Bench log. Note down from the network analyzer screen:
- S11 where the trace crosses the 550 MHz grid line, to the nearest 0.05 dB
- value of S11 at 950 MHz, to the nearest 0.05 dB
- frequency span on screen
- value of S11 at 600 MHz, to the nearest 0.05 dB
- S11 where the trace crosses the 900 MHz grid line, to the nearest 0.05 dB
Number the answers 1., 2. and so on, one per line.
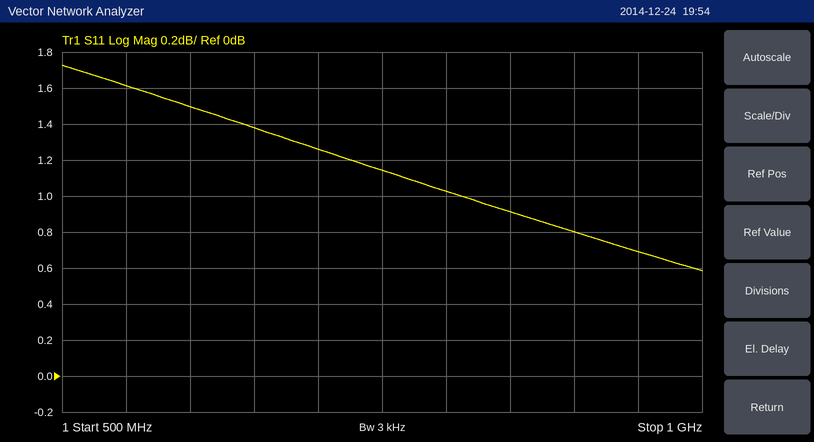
1. 1.60 dB
2. 0.70 dB
3. 500 MHz
4. 1.50 dB
5. 0.80 dB
